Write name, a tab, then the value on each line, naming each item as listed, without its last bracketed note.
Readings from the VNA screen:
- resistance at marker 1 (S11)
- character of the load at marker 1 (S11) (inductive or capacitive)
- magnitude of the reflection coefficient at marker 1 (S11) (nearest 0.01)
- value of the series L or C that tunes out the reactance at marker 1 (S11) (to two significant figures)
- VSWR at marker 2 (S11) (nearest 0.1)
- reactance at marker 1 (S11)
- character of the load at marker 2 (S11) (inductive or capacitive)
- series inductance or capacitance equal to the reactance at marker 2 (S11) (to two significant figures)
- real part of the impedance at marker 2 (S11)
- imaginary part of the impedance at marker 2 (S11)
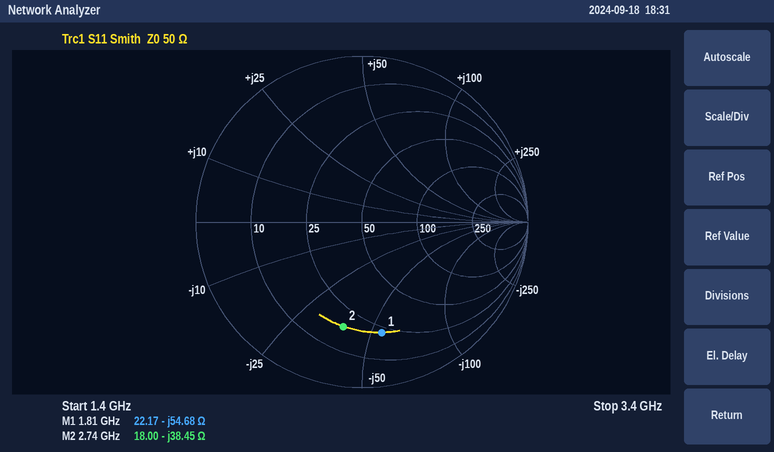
resistance at marker 1	22.17 Ω
character of the load at marker 1 (S11)	capacitive
magnitude of the reflection coefficient at marker 1 (S11)	0.68
value of the series L or C that tunes out the reactance at marker 1 (S11)	4.8 nH
VSWR at marker 2 (S11)	4.6
reactance at marker 1	-54.68 Ω
character of the load at marker 2 (S11)	capacitive
series inductance or capacitance equal to the reactance at marker 2 (S11)	1.5 pF
real part of the impedance at marker 2	18.00 Ω
imaginary part of the impedance at marker 2	-38.45 Ω
